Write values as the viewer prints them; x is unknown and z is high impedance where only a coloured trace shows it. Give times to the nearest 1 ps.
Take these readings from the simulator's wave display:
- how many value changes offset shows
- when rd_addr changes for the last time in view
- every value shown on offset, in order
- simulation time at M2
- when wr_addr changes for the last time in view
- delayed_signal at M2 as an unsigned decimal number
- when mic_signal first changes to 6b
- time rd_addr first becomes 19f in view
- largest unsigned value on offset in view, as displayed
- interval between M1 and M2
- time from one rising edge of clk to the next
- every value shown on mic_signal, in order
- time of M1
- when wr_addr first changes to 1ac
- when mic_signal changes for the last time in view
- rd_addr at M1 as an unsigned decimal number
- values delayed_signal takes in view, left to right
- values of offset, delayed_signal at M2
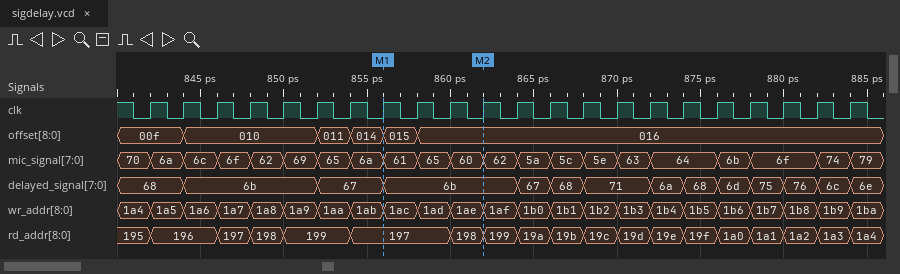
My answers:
5
884 ps
00f, 010, 011, 014, 015, 016
862 ps
884 ps
107
876 ps
874 ps
016
6 ps
2 ps
70, 6a, 6c, 6f, 62, 69, 65, 6a, 61, 65, 60, 62, 5a, 5c, 5e, 63, 64, 6b, 6f, 74, 79
856 ps
856 ps
884 ps
407
68, 6b, 67, 6b, 67, 68, 71, 6a, 68, 6d, 75, 76, 6c, 6e
offset=016, delayed_signal=6b
